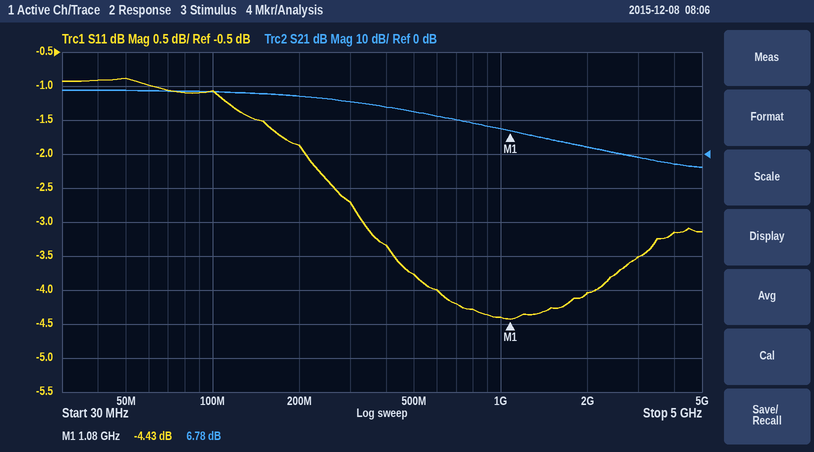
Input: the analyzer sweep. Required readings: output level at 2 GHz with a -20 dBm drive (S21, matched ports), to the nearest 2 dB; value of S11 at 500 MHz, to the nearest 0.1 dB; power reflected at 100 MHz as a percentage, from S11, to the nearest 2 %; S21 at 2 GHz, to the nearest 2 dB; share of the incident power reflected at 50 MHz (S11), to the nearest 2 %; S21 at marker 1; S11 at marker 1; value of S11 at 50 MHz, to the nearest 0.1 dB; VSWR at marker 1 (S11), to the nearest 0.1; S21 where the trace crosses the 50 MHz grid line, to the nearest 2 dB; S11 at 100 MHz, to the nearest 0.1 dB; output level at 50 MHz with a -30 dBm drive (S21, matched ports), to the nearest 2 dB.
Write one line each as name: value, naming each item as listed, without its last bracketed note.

output level at 2 GHz with a -20 dBm drive (S21, matched ports), to the nearest 2 dB: -18 dBm
value of S11 at 500 MHz, to the nearest 0.1 dB: -3.8 dB
power reflected at 100 MHz as a percentage, from S11, to the nearest 2 %: 78 %
S21 at 2 GHz, to the nearest 2 dB: 2 dB
share of the incident power reflected at 50 MHz (S11), to the nearest 2 %: 82 %
S21 at marker 1: 6.78 dB
S11 at marker 1: -4.43 dB
value of S11 at 50 MHz, to the nearest 0.1 dB: -0.9 dB
VSWR at marker 1 (S11), to the nearest 0.1: 4.0
S21 where the trace crosses the 50 MHz grid line, to the nearest 2 dB: 18 dB
S11 at 100 MHz, to the nearest 0.1 dB: -1.1 dB
output level at 50 MHz with a -30 dBm drive (S21, matched ports), to the nearest 2 dB: -12 dBm
